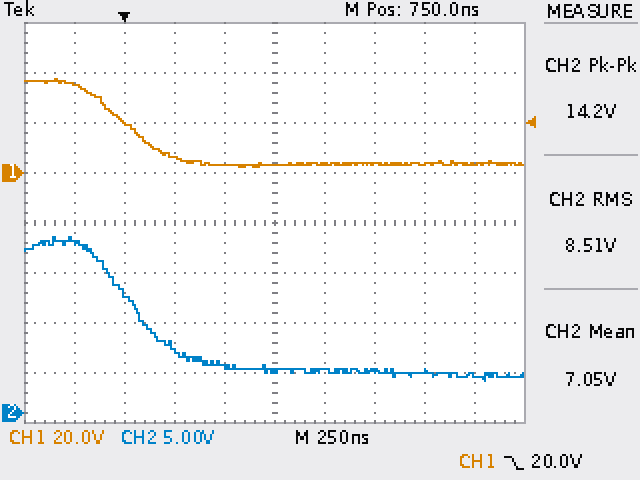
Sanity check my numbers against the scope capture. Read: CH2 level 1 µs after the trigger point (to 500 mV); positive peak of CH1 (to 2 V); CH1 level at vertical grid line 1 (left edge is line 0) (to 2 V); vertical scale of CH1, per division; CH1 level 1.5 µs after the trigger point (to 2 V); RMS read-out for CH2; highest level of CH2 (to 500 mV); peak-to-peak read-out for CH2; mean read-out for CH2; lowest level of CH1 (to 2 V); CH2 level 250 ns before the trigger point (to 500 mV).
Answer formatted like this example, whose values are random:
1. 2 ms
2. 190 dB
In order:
1. 4.5 V
2. 38 V
3. 36 V
4. 20 V
5. 4 V
6. 8.51 V
7. 17.5 V
8. 14.2 V
9. 7.05 V
10. 2 V
11. 17.0 V
